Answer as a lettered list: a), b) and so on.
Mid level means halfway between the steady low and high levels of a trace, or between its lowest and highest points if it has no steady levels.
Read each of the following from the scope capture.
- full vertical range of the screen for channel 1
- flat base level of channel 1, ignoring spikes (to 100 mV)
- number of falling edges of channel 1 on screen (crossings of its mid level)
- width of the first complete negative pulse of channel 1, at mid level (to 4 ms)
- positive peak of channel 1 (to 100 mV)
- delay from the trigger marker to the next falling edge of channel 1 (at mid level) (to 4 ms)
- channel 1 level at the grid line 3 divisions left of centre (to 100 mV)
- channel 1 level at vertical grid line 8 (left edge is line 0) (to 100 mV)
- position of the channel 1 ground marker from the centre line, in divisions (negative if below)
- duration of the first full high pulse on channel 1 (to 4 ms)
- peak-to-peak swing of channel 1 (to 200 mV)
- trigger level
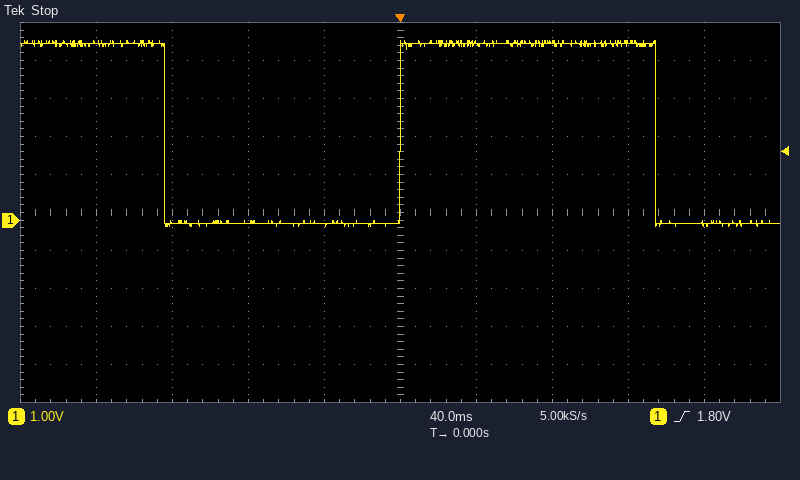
a) 10 V
b) -100 mV
c) 2
d) 124 ms
e) 4.7 V
f) 136 ms
g) -100 mV
h) 4.6 V
i) -0.2 div
j) 136 ms
k) 4.8 V
l) 1.80 V
